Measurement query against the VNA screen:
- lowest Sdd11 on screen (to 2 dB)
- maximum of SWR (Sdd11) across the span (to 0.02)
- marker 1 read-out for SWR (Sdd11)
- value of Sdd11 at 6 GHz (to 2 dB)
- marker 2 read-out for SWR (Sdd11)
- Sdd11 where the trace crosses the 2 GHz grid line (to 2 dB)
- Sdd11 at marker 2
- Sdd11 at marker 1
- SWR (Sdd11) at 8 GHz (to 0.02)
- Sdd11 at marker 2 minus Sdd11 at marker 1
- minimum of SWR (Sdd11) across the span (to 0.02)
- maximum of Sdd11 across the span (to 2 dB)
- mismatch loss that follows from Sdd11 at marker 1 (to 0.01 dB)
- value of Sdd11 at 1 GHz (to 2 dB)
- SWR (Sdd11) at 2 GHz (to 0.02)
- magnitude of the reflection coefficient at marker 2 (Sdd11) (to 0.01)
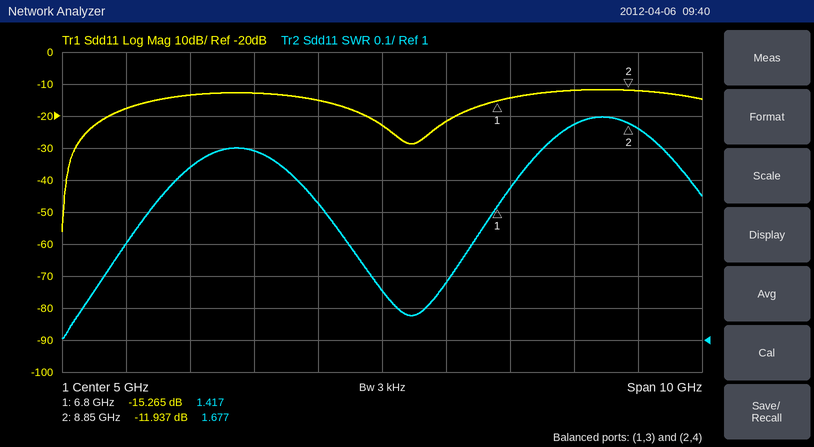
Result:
-56 dB
1.70
1.417
-22 dB
1.677
-14 dB
-11.937 dB
-15.265 dB
1.68
3.328 dB
1.00
-12 dB
0.13 dB
-18 dB
1.54
0.25
